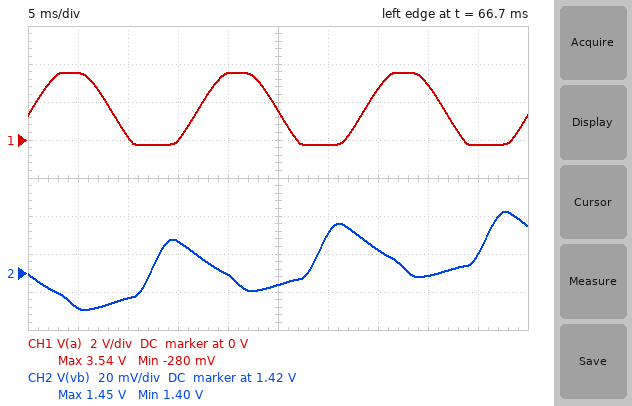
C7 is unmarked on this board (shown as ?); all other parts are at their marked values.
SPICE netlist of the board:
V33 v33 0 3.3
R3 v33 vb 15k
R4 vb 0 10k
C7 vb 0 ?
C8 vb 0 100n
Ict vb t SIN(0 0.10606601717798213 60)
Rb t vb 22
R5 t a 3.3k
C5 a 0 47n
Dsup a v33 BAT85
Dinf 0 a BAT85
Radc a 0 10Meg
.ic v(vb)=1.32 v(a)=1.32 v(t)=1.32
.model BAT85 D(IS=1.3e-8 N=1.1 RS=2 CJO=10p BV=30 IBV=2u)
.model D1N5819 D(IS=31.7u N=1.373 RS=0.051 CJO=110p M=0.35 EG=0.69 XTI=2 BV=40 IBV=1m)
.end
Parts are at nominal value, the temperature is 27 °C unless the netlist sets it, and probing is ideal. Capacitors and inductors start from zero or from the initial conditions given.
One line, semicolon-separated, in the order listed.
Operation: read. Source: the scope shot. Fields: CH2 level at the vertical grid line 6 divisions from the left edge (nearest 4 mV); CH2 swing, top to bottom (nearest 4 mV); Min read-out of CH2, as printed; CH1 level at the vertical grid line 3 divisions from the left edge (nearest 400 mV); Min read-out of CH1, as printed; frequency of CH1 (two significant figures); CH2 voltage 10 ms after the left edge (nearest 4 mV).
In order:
1.440 V; 52 mV; 1.40 V; 0 V; -280 mV; 60 Hz; 1.408 V
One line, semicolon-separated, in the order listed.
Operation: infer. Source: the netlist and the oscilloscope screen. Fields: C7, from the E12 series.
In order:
15 µF
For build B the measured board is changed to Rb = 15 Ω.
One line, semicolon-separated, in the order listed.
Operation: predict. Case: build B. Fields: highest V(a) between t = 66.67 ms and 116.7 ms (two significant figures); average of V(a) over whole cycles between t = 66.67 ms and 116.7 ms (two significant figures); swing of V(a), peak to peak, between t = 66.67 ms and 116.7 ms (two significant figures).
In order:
2.9 V; 1.3 V; 3.1 V
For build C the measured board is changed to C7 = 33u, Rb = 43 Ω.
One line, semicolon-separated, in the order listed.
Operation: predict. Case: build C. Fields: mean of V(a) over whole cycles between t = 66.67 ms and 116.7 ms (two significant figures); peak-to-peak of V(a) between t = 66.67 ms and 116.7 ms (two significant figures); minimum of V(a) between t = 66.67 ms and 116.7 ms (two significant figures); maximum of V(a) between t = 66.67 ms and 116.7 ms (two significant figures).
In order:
1.6 V; 3.9 V; -320 mV; 3.6 V
